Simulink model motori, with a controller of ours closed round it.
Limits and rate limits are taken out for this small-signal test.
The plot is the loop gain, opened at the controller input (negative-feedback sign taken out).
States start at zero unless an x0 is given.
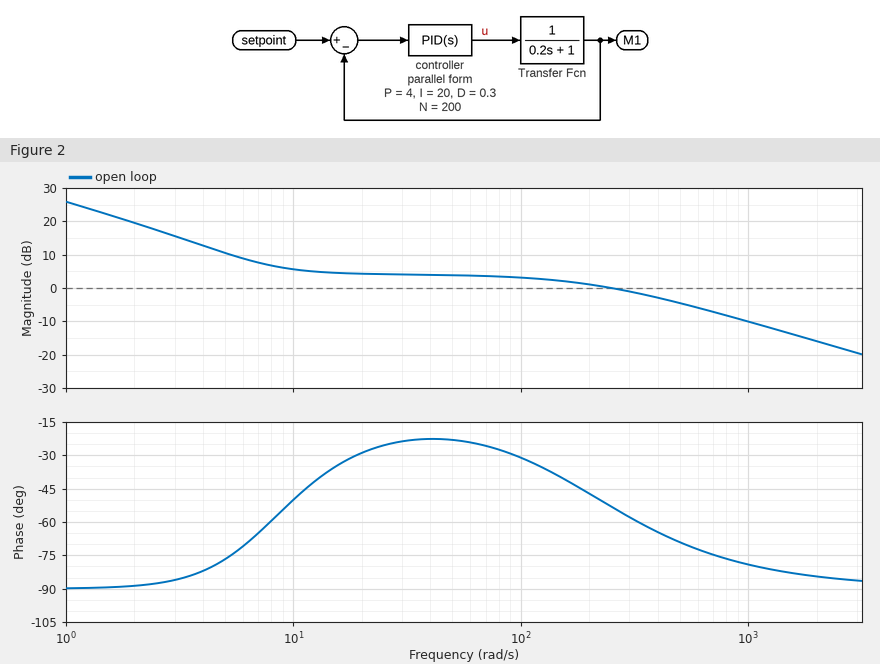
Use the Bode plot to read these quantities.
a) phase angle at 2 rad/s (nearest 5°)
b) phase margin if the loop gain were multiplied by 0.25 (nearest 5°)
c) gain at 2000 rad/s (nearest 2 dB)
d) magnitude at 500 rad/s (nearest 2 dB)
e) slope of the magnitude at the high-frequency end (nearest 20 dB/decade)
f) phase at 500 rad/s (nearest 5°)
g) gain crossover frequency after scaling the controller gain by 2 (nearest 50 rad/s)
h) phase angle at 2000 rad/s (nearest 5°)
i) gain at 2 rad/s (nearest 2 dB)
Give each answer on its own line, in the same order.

-90°
100°
-16 dB
-4 dB
-20 dB/decade
-70°
600 rad/s
-85°
20 dB
